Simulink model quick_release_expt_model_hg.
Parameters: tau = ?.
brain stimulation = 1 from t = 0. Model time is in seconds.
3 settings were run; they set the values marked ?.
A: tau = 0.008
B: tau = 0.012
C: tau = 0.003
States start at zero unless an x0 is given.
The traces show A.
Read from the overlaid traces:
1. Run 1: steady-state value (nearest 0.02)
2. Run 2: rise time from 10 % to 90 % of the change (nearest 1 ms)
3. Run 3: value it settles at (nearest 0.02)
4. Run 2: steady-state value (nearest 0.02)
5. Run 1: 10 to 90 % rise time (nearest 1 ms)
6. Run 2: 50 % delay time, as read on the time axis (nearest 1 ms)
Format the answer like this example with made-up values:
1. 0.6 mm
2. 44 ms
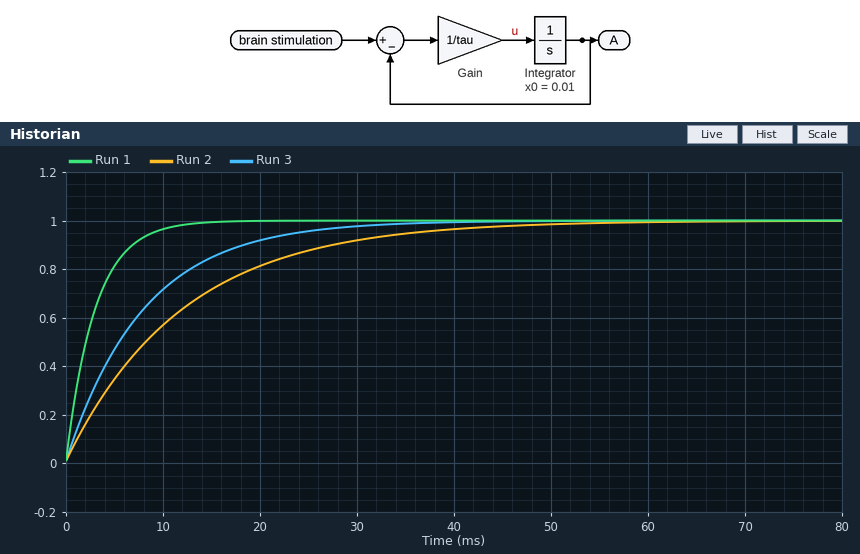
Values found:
1. 1.00
2. 26 ms
3. 1.00
4. 1.00
5. 7 ms
6. 8 ms
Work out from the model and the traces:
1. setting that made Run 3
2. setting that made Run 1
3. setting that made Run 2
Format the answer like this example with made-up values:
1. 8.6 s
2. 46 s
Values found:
1. A
2. C
3. B
